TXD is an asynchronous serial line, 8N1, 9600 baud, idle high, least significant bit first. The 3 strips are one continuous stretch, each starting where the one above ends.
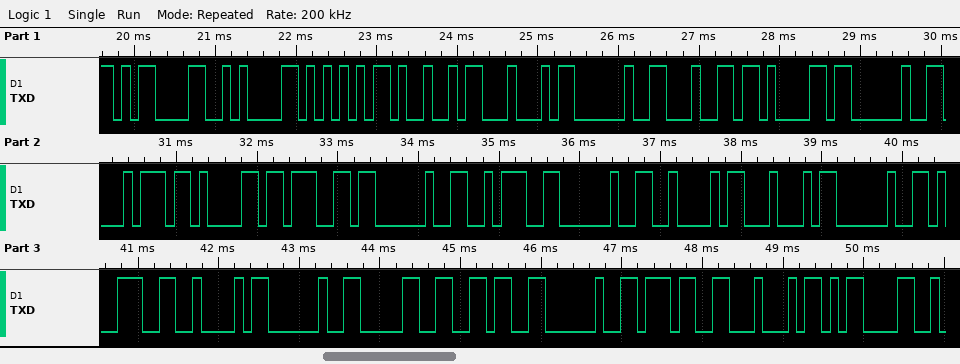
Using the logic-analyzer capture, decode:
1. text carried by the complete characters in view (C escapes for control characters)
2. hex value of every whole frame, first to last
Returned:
"\r\nUID da tag : BD 9B 06 7D\r"
0D 0A 55 49 44 20 64 61 20 74 61 67 20 3A 20 42 44 20 39 42 20 30 36 20 37 44 0D
